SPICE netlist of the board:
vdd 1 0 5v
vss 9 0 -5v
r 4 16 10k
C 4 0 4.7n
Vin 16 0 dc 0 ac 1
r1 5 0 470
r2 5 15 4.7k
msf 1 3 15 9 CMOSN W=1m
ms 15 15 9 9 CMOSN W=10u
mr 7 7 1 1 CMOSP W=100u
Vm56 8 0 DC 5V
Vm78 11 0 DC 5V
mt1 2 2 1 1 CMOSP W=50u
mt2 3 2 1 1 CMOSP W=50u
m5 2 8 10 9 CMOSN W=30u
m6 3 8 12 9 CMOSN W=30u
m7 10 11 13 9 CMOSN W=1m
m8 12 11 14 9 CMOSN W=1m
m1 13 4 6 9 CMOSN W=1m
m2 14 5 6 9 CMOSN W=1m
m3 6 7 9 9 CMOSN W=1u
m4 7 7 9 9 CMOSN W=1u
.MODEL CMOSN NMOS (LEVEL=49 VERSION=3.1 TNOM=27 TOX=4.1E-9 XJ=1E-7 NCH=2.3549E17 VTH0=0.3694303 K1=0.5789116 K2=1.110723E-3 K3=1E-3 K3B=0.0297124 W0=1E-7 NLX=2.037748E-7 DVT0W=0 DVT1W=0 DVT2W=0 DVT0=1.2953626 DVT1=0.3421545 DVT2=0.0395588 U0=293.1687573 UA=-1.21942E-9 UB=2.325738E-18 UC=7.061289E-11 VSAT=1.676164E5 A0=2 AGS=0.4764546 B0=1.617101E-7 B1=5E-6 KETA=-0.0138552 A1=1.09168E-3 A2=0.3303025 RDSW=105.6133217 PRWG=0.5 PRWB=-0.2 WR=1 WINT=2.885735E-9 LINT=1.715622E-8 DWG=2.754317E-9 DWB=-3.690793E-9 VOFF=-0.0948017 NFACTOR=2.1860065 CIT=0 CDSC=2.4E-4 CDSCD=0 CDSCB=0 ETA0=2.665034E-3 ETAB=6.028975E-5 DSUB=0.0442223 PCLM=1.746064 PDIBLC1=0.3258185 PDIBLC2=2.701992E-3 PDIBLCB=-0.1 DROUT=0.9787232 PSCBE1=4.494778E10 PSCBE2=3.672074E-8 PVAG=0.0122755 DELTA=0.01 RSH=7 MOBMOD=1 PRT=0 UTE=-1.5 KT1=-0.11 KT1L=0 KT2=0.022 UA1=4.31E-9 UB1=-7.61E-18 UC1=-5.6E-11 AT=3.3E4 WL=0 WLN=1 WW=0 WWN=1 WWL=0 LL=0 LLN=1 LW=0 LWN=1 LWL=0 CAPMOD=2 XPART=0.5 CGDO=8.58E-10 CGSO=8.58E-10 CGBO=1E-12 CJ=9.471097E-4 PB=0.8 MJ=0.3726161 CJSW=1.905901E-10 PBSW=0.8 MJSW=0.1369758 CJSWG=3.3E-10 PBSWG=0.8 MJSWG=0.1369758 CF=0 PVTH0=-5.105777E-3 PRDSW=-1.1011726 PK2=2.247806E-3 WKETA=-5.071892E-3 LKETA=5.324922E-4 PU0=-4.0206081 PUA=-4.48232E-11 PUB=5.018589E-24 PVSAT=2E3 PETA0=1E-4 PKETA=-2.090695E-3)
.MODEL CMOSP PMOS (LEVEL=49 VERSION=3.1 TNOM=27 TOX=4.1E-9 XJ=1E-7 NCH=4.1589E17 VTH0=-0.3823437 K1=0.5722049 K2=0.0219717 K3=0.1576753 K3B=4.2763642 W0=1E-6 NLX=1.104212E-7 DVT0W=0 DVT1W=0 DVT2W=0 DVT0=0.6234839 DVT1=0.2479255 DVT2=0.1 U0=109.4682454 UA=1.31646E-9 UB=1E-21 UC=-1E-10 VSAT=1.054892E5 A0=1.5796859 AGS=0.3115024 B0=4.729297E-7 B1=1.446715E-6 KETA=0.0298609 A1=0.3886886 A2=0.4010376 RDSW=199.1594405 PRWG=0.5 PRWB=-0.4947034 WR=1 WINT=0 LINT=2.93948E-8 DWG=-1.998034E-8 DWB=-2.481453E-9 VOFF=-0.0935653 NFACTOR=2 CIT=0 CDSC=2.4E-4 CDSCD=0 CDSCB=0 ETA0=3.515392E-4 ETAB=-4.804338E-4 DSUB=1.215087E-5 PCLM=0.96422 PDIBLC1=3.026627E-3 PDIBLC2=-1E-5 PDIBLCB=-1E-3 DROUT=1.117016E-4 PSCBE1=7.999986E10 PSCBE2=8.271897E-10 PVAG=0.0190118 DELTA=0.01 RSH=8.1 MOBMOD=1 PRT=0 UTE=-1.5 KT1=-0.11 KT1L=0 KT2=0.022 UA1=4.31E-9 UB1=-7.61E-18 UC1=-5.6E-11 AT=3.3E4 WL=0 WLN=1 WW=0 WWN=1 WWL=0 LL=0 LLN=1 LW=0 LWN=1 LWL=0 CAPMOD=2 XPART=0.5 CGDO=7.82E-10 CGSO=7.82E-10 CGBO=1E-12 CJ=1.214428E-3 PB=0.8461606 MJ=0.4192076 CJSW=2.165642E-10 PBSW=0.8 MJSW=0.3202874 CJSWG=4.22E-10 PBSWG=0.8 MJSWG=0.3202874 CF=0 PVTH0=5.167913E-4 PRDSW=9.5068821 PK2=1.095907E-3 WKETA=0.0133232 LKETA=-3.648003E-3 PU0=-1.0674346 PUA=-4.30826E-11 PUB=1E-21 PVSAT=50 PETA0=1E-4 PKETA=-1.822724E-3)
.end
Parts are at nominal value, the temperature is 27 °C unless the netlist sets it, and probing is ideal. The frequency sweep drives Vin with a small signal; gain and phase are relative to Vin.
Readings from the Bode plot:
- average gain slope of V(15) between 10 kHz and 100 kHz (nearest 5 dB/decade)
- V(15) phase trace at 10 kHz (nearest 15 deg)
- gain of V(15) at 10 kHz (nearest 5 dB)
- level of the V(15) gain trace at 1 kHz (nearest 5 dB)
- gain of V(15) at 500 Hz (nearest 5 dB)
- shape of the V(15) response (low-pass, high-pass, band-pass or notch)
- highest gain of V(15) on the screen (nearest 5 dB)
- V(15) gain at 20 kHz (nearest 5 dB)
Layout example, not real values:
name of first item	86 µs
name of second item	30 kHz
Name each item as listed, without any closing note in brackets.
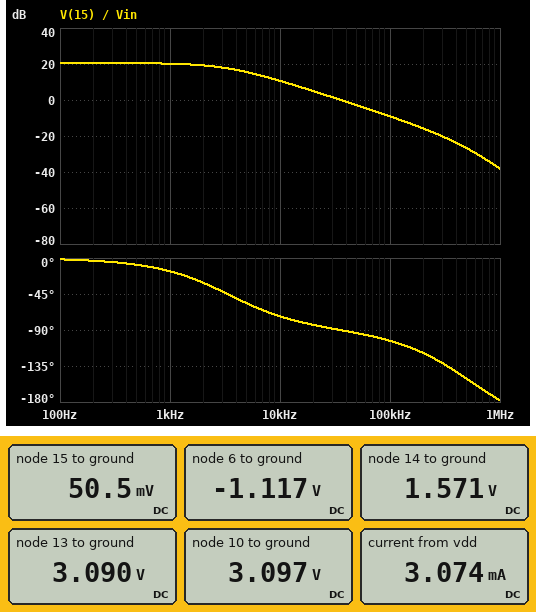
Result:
average gain slope of V(15) between 10 kHz and 100 kHz	-20 dB/decade
V(15) phase trace at 10 kHz	-75 deg
gain of V(15) at 10 kHz	10 dB
level of the V(15) gain trace at 1 kHz	20 dB
gain of V(15) at 500 Hz	20 dB
shape of the V(15) response	low-pass
highest gain of V(15) on the screen	20 dB
V(15) gain at 20 kHz	5 dB
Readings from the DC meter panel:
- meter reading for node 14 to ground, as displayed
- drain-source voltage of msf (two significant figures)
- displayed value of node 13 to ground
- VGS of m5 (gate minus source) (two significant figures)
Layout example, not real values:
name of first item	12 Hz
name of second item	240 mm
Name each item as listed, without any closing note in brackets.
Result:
meter reading for node 14 to ground, as displayed	1.571 V
drain-source voltage of msf	4.9 V
displayed value of node 13 to ground	3.090 V
VGS of m5 (gate minus source)	1.9 V
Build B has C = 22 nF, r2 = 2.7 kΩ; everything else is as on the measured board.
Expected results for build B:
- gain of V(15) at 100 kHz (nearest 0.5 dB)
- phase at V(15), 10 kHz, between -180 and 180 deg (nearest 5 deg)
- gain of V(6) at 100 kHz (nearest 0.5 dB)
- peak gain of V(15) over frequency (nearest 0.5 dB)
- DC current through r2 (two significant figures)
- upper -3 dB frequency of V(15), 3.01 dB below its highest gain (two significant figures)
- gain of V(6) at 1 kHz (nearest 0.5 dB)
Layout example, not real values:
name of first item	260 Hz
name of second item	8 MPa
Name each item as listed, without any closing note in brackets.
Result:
gain of V(15) at 100 kHz	-26.5 dB
phase at V(15), 10 kHz, between -180 and 180 deg	-85 deg
gain of V(6) at 100 kHz	-44.0 dB
peak gain of V(15) over frequency	16.5 dB
DC current through r2	9.9 µA
upper -3 dB frequency of V(15), 3.01 dB below its highest gain	720 Hz
gain of V(6) at 1 kHz	-6.0 dB
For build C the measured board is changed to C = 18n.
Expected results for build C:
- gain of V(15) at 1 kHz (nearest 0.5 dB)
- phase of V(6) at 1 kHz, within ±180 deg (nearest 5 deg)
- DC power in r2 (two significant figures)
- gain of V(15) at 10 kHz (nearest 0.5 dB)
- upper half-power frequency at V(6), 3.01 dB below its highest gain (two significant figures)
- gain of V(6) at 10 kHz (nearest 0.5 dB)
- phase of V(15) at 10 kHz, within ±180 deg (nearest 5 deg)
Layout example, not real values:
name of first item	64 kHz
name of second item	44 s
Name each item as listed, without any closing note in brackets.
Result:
gain of V(15) at 1 kHz	17.0 dB
phase of V(6) at 1 kHz, within ±180 deg	-50 deg
DC power in r2	450 nW
gain of V(15) at 10 kHz	-0.5 dB
upper half-power frequency at V(6), 3.01 dB below its highest gain	880 Hz
gain of V(6) at 10 kHz	-22.5 dB
phase of V(15) at 10 kHz, within ±180 deg	-85 deg
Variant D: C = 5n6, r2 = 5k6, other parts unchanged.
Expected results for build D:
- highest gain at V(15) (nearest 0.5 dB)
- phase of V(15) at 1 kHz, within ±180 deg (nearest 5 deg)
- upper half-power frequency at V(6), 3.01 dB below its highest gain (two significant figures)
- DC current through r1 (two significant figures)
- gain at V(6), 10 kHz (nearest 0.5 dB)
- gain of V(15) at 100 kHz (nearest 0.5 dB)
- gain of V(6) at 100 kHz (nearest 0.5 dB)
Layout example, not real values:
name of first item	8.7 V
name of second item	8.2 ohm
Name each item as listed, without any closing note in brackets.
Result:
highest gain at V(15)	22.0 dB
phase of V(15) at 1 kHz, within ±180 deg	-20 deg
upper half-power frequency at V(6), 3.01 dB below its highest gain	2.8 kHz
DC current through r1	9.7 µA
gain at V(6), 10 kHz	-12.5 dB
gain of V(15) at 100 kHz	-9.5 dB
gain of V(6) at 100 kHz	-32.5 dB
